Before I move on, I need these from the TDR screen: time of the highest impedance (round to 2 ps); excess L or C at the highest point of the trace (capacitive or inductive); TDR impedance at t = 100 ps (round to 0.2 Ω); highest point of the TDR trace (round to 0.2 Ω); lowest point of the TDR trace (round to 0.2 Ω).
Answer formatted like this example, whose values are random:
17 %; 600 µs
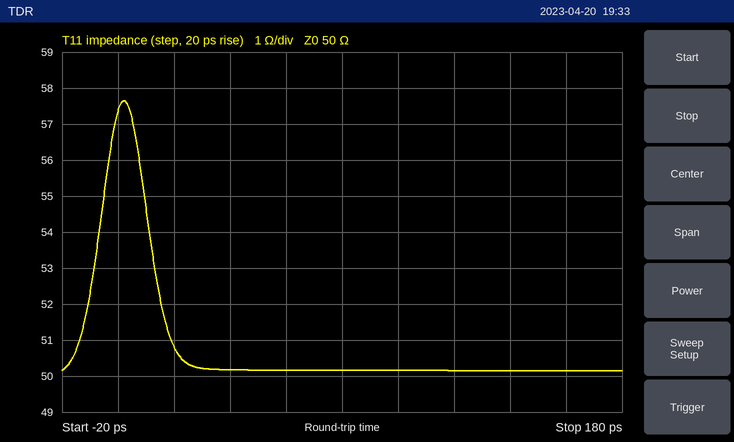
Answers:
2 ps; inductive; 50.2 Ω; 57.6 Ω; 50.2 Ω
